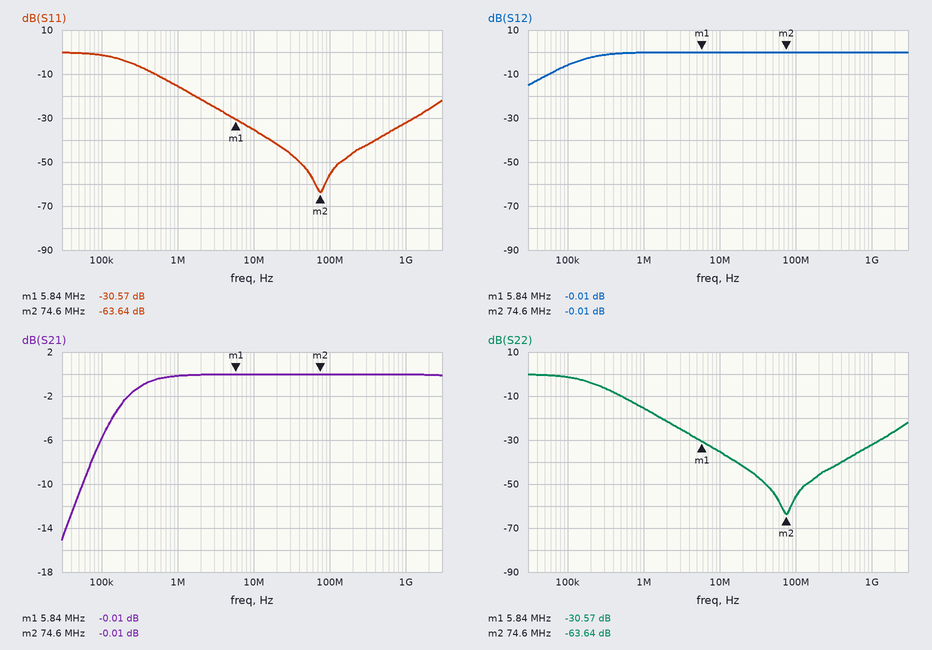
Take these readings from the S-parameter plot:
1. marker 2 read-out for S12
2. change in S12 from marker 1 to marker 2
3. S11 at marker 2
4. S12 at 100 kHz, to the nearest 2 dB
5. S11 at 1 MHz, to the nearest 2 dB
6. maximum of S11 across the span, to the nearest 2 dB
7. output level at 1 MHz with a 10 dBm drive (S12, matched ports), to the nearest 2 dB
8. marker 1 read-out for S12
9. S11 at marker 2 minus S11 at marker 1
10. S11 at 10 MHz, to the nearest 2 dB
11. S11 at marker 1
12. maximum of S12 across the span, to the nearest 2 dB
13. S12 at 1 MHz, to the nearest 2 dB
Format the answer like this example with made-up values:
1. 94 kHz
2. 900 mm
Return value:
1. -0.01 dB
2. 0.00 dB
3. -63.64 dB
4. -6 dB
5. -16 dB
6. 0 dB
7. 10 dBm
8. -0.01 dB
9. -33.07 dB
10. -36 dB
11. -30.57 dB
12. 0 dB
13. 0 dB
